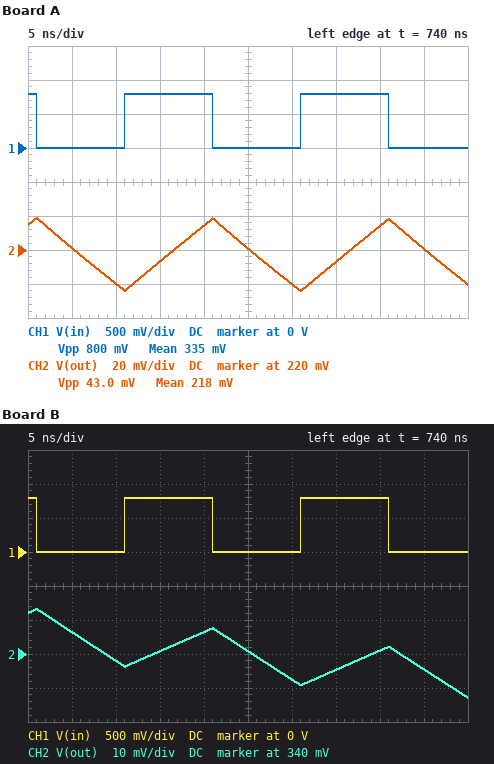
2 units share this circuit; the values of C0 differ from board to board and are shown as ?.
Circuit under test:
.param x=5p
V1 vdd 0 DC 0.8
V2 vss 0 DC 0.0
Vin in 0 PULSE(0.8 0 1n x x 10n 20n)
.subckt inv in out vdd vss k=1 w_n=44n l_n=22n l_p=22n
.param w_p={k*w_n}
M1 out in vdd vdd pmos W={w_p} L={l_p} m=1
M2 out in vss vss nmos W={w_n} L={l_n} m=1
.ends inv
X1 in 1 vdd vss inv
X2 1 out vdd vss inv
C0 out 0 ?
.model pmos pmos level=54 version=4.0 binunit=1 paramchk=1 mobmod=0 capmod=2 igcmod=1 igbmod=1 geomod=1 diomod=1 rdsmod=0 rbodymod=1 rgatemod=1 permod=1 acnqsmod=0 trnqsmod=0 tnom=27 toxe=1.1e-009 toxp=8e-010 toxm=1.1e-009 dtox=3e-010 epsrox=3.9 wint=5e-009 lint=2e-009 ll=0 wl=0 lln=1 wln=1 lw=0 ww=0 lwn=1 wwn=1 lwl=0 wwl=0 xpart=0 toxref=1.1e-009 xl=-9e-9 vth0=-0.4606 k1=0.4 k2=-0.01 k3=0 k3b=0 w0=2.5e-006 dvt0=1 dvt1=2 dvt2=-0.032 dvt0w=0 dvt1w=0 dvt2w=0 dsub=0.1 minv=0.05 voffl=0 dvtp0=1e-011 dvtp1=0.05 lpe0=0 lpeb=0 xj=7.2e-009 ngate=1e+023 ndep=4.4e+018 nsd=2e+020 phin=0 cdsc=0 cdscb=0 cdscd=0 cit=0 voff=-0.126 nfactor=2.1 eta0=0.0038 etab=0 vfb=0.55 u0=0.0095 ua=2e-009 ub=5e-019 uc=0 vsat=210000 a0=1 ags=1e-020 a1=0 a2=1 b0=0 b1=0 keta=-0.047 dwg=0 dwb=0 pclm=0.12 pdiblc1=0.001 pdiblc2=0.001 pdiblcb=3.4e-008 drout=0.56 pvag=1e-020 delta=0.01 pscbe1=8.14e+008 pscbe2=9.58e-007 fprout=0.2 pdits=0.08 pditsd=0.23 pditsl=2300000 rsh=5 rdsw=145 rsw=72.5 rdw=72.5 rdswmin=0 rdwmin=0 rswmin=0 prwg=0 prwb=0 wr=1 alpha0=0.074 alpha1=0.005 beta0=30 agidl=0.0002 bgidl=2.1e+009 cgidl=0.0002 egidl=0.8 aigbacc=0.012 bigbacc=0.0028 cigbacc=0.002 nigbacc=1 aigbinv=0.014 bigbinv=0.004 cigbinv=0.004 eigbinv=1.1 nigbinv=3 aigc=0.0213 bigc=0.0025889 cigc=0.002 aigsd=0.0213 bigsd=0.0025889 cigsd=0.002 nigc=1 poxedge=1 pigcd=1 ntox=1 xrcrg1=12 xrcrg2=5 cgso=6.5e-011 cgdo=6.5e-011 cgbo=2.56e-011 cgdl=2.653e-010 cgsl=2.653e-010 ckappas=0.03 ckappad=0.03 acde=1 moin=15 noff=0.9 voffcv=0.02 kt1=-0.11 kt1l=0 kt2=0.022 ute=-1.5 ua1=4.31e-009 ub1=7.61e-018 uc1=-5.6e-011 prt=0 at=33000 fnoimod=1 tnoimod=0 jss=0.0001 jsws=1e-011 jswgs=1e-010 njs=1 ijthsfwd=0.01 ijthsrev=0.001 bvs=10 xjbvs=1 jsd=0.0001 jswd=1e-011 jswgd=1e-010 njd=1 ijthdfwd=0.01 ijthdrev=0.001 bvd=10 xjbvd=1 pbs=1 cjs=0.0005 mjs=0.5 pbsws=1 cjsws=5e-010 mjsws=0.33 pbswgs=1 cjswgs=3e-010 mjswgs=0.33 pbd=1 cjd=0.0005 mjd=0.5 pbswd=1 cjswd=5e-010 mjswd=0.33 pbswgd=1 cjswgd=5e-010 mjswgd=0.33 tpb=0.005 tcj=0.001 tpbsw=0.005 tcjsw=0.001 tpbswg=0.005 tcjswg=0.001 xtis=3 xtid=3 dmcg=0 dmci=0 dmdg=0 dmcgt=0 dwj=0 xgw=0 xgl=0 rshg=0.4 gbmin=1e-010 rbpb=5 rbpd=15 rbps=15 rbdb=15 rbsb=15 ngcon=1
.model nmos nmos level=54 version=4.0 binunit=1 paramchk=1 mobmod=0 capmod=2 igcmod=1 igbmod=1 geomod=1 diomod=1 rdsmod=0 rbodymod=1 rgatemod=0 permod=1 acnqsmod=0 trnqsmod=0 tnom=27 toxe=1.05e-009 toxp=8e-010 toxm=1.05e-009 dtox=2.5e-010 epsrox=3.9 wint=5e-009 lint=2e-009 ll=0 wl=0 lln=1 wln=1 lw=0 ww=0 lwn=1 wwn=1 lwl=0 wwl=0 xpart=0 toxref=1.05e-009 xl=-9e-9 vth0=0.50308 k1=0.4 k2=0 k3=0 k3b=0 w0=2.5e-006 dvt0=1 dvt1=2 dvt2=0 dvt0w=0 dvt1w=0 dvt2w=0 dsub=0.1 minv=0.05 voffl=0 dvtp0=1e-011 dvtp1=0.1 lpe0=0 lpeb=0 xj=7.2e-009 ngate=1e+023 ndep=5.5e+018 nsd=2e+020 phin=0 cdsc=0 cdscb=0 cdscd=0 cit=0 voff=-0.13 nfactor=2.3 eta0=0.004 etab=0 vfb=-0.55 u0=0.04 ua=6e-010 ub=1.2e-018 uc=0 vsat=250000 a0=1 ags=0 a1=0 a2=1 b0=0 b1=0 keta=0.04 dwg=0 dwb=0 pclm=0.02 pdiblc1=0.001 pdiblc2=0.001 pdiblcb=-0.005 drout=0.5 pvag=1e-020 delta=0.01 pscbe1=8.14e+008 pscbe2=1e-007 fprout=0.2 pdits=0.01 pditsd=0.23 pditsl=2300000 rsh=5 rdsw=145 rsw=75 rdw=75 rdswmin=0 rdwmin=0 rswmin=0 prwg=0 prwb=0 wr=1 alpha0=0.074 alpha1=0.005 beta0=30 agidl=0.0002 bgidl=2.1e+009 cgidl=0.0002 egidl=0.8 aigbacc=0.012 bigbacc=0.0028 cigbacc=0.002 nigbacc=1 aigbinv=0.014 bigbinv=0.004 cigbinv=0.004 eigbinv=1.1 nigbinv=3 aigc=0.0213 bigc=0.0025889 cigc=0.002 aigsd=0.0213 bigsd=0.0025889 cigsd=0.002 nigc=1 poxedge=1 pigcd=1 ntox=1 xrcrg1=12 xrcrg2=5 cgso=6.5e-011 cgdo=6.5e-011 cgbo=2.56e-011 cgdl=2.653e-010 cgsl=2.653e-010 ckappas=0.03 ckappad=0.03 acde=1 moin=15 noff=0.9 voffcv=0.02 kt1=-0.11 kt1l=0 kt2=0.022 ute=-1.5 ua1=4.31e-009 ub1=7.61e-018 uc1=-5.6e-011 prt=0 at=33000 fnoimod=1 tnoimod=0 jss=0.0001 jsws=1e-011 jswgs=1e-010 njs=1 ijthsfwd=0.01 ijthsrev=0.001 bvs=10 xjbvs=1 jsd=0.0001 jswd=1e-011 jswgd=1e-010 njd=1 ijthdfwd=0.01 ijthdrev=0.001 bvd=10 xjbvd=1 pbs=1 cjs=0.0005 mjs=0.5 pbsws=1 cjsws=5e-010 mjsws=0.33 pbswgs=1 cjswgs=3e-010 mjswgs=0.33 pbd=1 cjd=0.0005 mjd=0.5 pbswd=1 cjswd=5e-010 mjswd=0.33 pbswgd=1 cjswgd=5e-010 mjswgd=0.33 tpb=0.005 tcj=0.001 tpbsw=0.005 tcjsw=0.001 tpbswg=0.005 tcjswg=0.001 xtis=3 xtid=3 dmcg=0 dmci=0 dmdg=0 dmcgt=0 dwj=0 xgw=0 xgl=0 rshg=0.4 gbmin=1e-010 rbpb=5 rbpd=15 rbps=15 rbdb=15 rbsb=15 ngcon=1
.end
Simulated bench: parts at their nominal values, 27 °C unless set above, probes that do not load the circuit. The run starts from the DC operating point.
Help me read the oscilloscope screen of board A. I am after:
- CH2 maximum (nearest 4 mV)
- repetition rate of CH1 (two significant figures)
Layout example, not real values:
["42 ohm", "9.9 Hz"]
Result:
["240 mV", "50 MHz"]
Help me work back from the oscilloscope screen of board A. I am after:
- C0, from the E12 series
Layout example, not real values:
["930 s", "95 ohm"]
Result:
["6.8 pF"]
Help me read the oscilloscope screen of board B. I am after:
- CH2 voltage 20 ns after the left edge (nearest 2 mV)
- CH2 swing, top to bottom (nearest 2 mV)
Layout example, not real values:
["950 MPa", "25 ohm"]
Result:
["346 mV", "26 mV"]
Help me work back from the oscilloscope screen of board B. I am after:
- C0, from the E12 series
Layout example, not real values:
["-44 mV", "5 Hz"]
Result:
["22 pF"]
